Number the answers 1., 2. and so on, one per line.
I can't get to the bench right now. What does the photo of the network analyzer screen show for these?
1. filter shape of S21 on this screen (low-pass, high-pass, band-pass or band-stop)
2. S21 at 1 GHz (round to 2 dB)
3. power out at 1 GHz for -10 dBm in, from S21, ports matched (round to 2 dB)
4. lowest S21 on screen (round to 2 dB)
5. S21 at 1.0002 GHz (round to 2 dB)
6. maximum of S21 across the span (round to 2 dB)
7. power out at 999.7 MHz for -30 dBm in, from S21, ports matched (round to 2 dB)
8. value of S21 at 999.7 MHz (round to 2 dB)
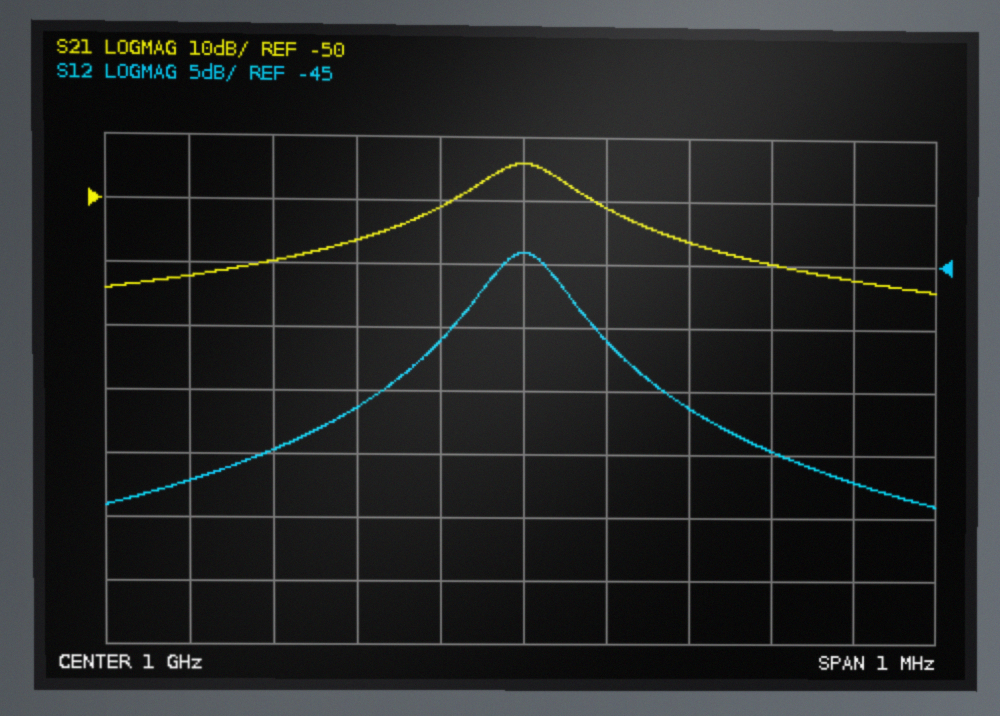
1. band-pass
2. -44 dB
3. -54 dBm
4. -64 dB
5. -56 dB
6. -44 dB
7. -90 dBm
8. -60 dB
